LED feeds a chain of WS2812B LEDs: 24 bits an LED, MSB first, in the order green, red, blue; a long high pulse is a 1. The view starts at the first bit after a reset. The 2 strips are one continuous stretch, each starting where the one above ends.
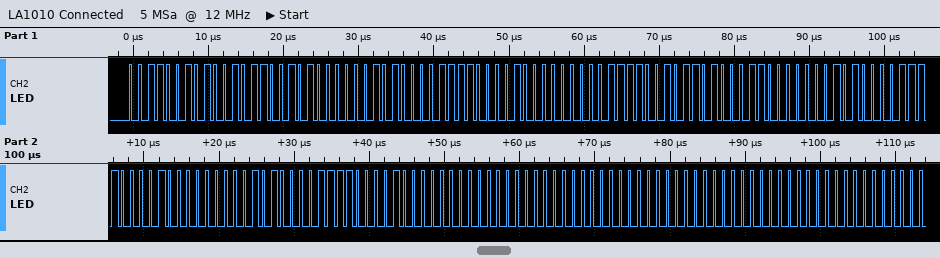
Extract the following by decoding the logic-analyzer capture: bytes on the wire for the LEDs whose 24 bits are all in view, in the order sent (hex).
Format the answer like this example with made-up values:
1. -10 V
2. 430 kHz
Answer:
1. 32 96 50 28 78 40 1E 5A 30 14 3C 20 0A 1E 10 00 00 00 00 00 00
